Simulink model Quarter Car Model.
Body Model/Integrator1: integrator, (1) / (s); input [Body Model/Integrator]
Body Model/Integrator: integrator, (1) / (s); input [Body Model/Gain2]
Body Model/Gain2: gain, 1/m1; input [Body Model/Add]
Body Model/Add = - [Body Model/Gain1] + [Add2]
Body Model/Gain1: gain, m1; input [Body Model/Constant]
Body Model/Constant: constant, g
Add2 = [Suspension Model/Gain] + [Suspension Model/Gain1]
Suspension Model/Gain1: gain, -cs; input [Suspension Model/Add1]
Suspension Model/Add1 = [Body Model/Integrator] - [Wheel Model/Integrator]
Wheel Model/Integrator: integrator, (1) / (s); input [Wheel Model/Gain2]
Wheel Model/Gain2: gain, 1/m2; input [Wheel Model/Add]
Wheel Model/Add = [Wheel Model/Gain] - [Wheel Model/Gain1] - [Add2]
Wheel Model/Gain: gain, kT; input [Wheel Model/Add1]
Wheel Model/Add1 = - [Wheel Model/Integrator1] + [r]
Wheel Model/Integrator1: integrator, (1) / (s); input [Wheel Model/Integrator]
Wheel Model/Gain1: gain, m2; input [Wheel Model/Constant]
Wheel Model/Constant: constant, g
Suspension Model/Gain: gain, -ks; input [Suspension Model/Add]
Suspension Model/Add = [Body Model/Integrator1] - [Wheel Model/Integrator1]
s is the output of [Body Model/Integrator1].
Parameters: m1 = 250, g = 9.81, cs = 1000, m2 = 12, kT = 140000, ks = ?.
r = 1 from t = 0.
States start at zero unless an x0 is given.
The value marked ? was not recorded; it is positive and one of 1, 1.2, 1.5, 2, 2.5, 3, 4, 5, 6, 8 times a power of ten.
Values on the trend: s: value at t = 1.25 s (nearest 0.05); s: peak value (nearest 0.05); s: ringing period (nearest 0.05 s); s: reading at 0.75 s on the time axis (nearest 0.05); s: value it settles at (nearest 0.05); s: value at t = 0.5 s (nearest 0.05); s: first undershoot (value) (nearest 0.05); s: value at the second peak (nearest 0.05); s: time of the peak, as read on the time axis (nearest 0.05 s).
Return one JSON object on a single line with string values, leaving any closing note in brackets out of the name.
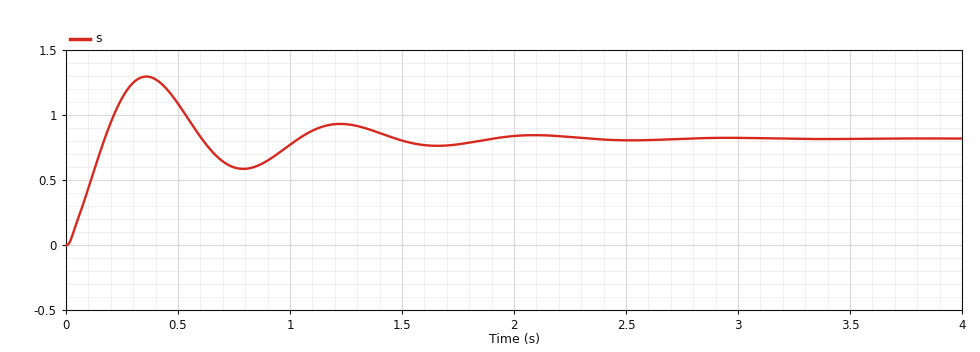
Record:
{"s: value at t = 1.25 s": "0.95", "s: peak value": "1.30", "s: ringing period": "0.85 s", "s: reading at 0.75 s on the time axis": "0.60", "s: value it settles at": "0.80", "s: value at t = 0.5 s": "1.10", "s: first undershoot (value)": "0.60", "s: value at the second peak": "0.95", "s: time of the peak, as read on the time axis": "0.35 s"}
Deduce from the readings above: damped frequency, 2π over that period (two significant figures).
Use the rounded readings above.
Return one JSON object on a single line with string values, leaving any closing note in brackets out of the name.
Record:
{"damped frequency, 2π over that period": "7.4 rad/s"}
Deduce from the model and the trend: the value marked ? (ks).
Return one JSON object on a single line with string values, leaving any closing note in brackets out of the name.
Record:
{"the value marked ?": "15000"}
